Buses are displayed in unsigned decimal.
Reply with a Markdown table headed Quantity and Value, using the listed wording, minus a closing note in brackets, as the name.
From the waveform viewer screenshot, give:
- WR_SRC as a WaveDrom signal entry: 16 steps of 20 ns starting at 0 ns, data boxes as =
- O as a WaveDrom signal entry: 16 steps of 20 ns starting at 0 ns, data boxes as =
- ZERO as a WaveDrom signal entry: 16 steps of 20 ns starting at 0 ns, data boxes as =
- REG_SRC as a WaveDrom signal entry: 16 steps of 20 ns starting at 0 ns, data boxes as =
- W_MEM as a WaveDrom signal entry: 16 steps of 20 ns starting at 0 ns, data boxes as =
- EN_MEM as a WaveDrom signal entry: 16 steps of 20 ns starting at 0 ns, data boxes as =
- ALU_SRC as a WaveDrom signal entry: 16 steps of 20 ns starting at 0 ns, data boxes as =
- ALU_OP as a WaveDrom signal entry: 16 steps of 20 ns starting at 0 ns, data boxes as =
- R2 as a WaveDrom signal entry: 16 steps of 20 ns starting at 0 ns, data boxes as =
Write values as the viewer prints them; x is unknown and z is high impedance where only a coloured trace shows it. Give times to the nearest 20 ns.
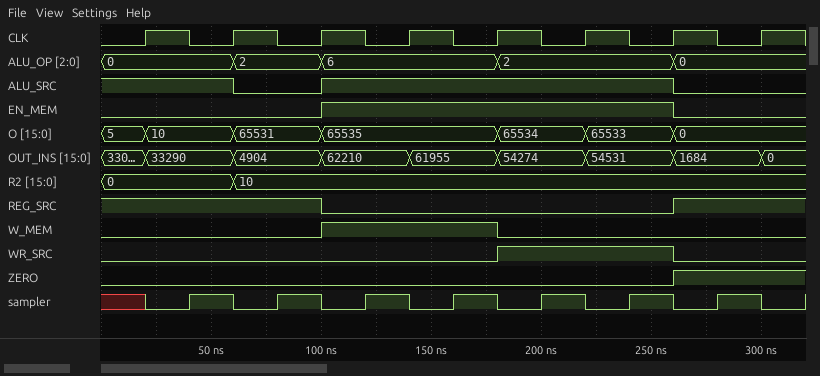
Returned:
| Quantity | Value |
|---|---|
| WR_SRC as a WaveDrom signal entry: 16 steps of 20 ns starting at 0 ns, data boxes as = | {name: 'WR_SRC', wave: '0........1...0..'} |
| O as a WaveDrom signal entry: 16 steps of 20 ns starting at 0 ns, data boxes as = | {name: 'O', wave: '==.=.=...=.=.=..', data: '5 10 65531 65535 65534 65533 0'} |
| ZERO as a WaveDrom signal entry: 16 steps of 20 ns starting at 0 ns, data boxes as = | {name: 'ZERO', wave: '0............1..'} |
| REG_SRC as a WaveDrom signal entry: 16 steps of 20 ns starting at 0 ns, data boxes as = | {name: 'REG_SRC', wave: '1....0.......1..'} |
| W_MEM as a WaveDrom signal entry: 16 steps of 20 ns starting at 0 ns, data boxes as = | {name: 'W_MEM', wave: '0....1...0......'} |
| EN_MEM as a WaveDrom signal entry: 16 steps of 20 ns starting at 0 ns, data boxes as = | {name: 'EN_MEM', wave: '0....1.......0..'} |
| ALU_SRC as a WaveDrom signal entry: 16 steps of 20 ns starting at 0 ns, data boxes as = | {name: 'ALU_SRC', wave: '1..0.1.......0..'} |
| ALU_OP as a WaveDrom signal entry: 16 steps of 20 ns starting at 0 ns, data boxes as = | {name: 'ALU_OP', wave: '=..=.=...=...=..', data: '0 2 6 2 0'} |
| R2 as a WaveDrom signal entry: 16 steps of 20 ns starting at 0 ns, data boxes as = | {name: 'R2', wave: '=..=............', data: '0 10'} |
